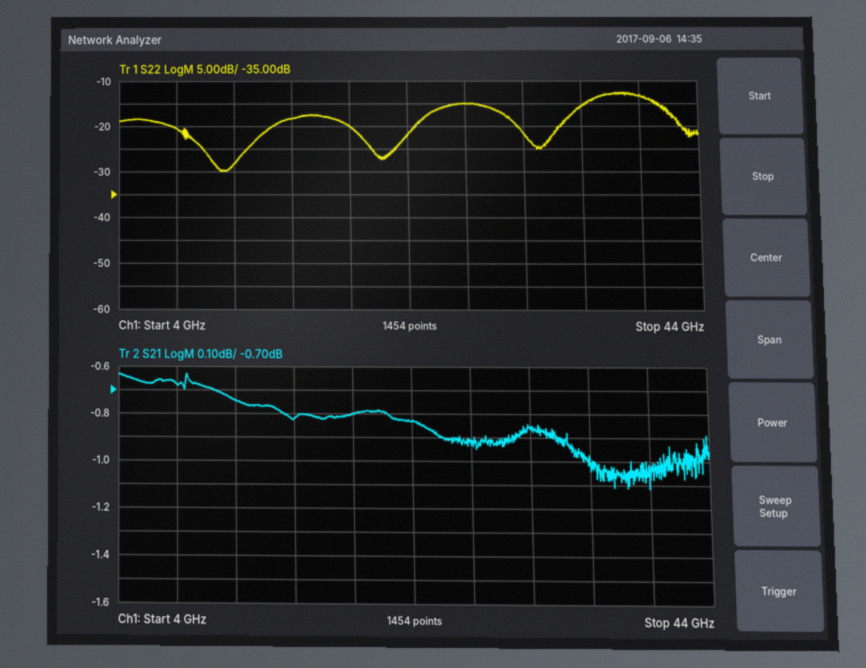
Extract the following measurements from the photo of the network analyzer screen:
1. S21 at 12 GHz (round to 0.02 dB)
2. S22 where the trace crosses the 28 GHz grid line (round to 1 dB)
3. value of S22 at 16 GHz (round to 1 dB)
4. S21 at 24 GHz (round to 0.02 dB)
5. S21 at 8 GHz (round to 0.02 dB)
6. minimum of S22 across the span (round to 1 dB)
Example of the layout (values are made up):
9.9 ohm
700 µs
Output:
-0.74 dB
-15 dB
-18 dB
-0.84 dB
-0.68 dB
-30 dB
